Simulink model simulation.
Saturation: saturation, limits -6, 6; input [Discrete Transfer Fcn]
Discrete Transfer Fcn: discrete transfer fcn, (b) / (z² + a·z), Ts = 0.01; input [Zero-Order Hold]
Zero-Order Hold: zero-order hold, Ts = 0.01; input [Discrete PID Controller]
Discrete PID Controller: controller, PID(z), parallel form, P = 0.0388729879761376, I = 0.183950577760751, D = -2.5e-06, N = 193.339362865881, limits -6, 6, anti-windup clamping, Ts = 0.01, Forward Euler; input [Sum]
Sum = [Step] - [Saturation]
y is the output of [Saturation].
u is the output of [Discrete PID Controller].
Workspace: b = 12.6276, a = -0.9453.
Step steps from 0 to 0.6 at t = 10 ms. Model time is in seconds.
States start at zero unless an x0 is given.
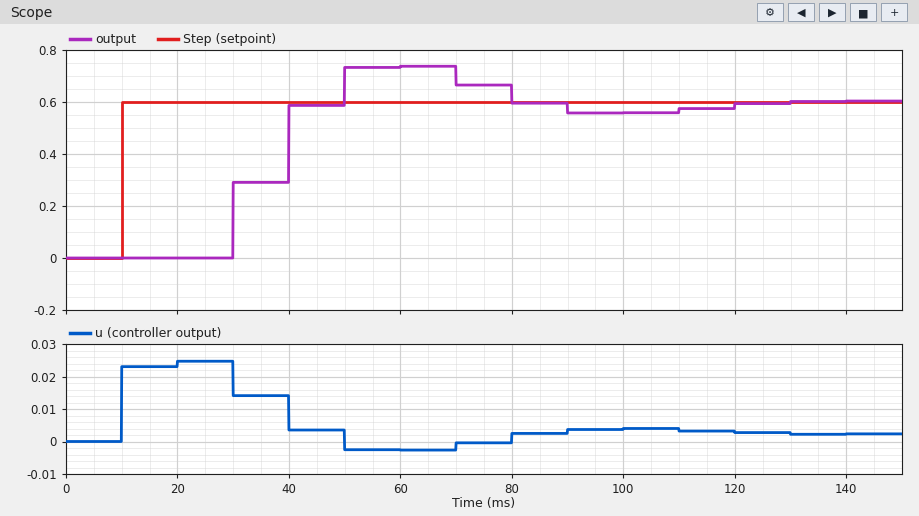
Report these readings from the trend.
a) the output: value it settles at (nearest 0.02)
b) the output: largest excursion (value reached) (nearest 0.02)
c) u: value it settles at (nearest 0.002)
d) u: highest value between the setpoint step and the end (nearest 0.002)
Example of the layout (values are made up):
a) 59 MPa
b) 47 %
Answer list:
a) 0.60
b) 0.74
c) 0.002
d) 0.024
